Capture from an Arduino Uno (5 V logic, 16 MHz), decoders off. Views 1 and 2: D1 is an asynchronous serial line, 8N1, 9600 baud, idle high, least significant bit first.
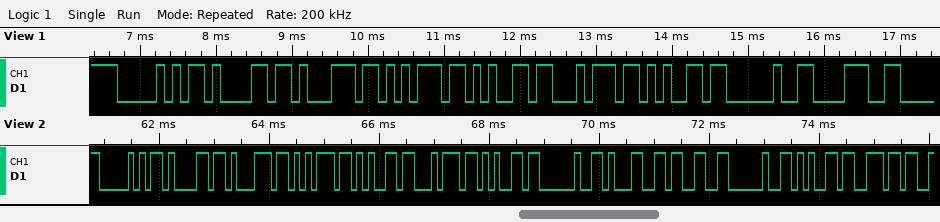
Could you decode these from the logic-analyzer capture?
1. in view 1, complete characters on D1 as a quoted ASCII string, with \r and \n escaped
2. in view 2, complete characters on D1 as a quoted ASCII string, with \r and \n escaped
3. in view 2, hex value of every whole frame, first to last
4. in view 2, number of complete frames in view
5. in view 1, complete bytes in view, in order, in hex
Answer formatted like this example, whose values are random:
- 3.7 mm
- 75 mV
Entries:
- "Paquete 8"
- "Paquete 13 en"
- 0x50 0x61 0x71 0x75 0x65 0x74 0x65 0x20 0x31 0x33 0x20 0x65 0x6E
- 13
- 0x50 0x61 0x71 0x75 0x65 0x74 0x65 0x20 0x38
